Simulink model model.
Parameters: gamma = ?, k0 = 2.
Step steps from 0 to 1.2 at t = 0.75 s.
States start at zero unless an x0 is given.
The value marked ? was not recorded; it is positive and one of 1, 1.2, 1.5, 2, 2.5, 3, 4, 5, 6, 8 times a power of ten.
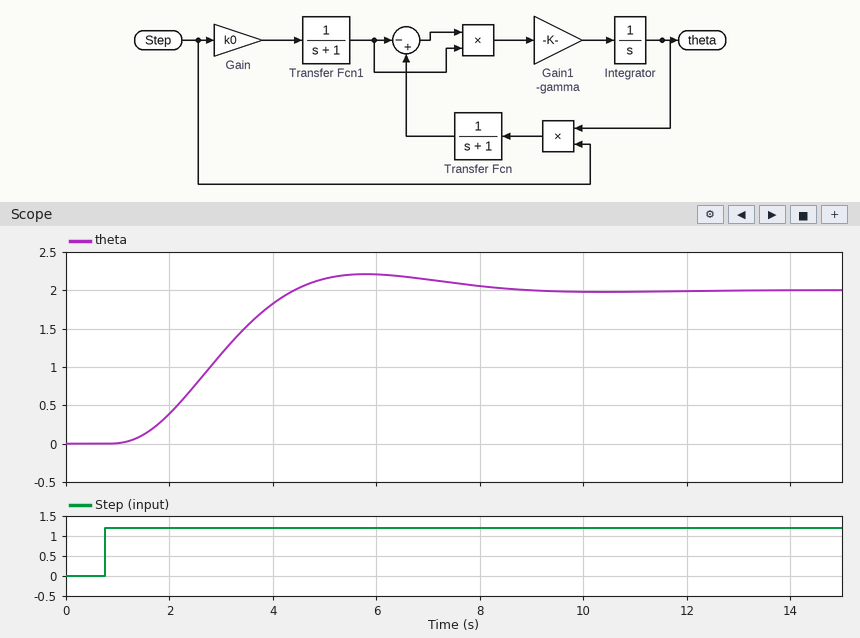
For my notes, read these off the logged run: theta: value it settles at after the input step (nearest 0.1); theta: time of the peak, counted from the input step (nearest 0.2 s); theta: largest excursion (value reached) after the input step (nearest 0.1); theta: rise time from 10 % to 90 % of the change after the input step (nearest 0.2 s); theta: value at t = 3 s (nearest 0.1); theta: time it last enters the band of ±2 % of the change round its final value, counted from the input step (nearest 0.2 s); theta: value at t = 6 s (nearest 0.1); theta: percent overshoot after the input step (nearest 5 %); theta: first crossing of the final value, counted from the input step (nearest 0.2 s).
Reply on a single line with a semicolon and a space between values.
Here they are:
2.0; 5.0 s; 2.2; 2.2 s; 1.2; 7.4 s; 2.2; 10 %; 3.6 s
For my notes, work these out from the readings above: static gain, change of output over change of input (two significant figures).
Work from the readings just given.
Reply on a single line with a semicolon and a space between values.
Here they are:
1.7
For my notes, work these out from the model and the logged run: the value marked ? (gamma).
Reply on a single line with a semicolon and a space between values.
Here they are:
0.25
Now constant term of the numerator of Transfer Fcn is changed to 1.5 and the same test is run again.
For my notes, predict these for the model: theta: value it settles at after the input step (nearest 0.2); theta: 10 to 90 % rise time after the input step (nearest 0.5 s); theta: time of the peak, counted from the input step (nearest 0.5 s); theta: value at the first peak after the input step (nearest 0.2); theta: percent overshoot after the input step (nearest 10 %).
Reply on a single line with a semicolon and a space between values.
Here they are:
1.4; 1.5 s; 4.0 s; 1.6; 20 %
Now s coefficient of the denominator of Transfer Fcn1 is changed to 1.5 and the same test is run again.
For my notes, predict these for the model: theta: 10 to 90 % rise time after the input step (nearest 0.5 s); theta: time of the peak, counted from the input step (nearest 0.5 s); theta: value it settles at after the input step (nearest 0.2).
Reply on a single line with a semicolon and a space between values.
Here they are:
3.0 s; 6.0 s; 2.0
